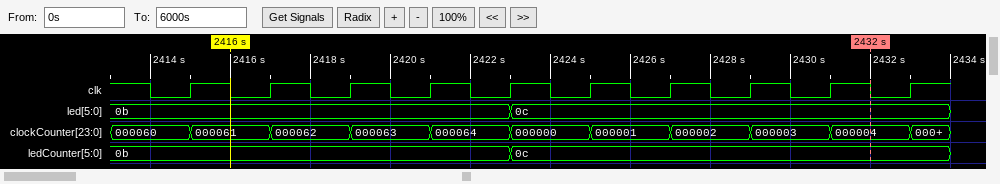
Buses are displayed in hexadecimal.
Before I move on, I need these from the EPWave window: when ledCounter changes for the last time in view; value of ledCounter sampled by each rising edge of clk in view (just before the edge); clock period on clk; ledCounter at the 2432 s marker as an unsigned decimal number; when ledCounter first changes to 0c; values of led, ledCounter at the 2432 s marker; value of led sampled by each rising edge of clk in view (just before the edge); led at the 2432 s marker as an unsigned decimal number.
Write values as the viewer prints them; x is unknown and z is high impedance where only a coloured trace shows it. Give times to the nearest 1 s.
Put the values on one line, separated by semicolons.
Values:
2423 s; 0b, 0b, 0b, 0b, 0b, 0c, 0c, 0c, 0c, 0c; 2 s; 12; 2423 s; led=0c, ledCounter=0c; 0b, 0b, 0b, 0b, 0b, 0c, 0c, 0c, 0c, 0c; 12
